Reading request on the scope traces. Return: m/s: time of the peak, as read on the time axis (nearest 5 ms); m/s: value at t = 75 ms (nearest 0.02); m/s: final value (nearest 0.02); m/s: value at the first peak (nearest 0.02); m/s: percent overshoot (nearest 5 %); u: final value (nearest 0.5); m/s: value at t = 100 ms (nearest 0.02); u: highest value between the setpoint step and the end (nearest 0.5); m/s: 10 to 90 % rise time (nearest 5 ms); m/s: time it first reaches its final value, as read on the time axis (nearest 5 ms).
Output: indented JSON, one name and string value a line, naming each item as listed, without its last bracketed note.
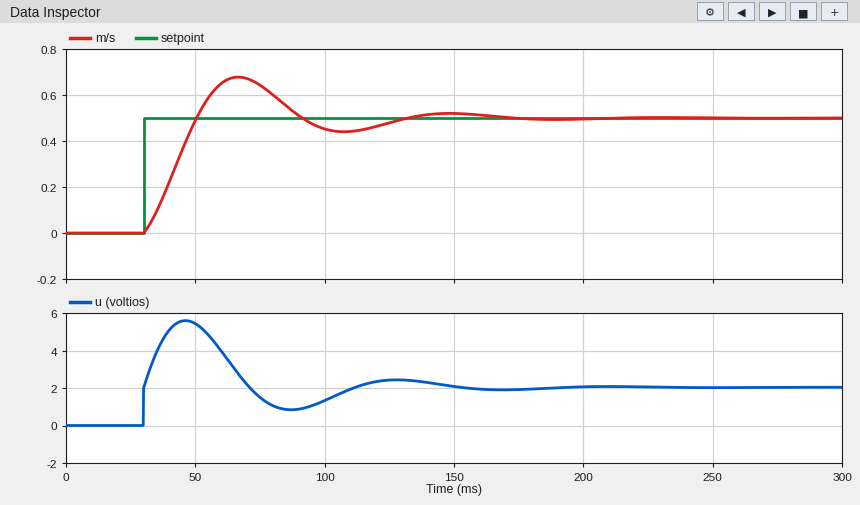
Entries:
{
  "m/s: time of the peak, as read on the time axis": "65 ms",
  "m/s: value at t = 75 ms": "0.64",
  "m/s: final value": "0.50",
  "m/s: value at the first peak": "0.68",
  "m/s: percent overshoot": "35 %",
  "u: final value": "2.0",
  "m/s: value at t = 100 ms": "0.46",
  "u: highest value between the setpoint step and the end": "5.5",
  "m/s: 10 to 90 % rise time": "15 ms",
  "m/s: time it first reaches its final value, as read on the time axis": "50 ms"
}
